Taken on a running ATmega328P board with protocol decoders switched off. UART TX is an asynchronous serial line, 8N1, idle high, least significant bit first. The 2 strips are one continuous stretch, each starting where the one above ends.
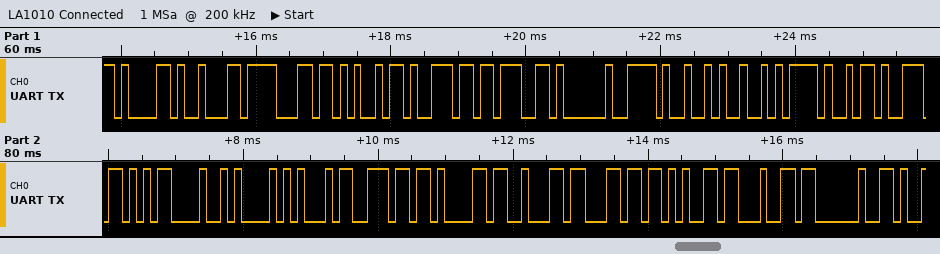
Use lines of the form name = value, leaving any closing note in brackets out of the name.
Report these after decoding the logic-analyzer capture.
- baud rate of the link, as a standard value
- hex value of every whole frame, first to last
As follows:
baud rate of the link, as a standard value = 9600 baud
hex value of every whole frame, first to last = 0x61 0x62 0x6C 0x69 0x6E 0x67 0x20 0x49 0x52 0x69 0x6E 0x0D 0x0A 0x45 0x6E 0x61 0x62 0x6C 0x65 0x64 0x20
